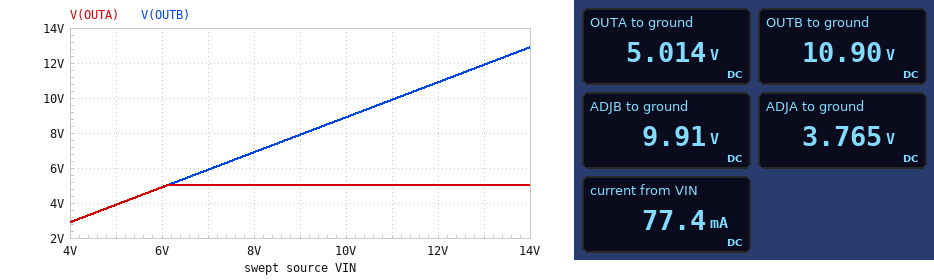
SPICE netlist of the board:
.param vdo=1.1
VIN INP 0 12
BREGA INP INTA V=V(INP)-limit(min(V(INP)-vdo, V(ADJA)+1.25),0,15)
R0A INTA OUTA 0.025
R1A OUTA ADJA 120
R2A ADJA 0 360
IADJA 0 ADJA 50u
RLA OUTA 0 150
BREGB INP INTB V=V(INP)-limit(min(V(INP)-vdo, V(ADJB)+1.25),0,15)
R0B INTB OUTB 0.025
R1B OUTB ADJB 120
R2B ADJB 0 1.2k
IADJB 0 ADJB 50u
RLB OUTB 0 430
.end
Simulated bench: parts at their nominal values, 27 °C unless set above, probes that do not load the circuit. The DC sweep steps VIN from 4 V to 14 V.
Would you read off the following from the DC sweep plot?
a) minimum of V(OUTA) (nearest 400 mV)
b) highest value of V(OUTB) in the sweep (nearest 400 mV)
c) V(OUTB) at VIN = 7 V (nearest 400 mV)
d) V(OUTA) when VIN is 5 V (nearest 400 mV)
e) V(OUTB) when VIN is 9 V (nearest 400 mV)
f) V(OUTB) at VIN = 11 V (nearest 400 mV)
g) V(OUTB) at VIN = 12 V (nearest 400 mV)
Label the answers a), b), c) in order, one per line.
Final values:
a) 2.8 V
b) 12.8 V
c) 6.0 V
d) 4.0 V
e) 8.0 V
f) 10.0 V
g) 10.8 V
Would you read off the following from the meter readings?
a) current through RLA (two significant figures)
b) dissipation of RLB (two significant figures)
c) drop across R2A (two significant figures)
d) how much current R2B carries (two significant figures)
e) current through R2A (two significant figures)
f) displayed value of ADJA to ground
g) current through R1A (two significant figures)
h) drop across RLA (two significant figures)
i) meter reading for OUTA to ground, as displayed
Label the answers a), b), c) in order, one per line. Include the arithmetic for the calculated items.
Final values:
a) (5.014 V) / 150 Ω = 33 mA
b) (10.9 V)^2 / 430 Ω = 280 mW
c) 3.765 V = 3.8 V
d) (9.91 V) / 1.2 kΩ = 8.3 mA
e) (3.765 V) / 360 Ω = 10 mA
f) 3.765 V
g) (5.014 V - 3.765 V) / 120 Ω = 10 mA
h) 5.014 V = 5.0 V
i) 5.014 V
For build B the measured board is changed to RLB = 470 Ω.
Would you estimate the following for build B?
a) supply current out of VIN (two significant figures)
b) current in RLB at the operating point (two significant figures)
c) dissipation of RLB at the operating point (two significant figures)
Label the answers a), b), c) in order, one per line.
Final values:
a) 75 mA
b) 23 mA
c) 250 mW
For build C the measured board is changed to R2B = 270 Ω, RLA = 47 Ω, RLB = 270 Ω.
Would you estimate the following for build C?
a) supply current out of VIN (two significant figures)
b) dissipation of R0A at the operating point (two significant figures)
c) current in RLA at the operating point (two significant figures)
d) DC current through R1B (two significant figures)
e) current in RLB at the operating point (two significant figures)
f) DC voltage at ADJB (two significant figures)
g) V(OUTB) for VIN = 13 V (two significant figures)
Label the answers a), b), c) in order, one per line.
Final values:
a) 140 mA
b) 340 µW
c) 110 mA
d) 10 mA
e) 15 mA
f) 2.8 V
g) 4.1 V
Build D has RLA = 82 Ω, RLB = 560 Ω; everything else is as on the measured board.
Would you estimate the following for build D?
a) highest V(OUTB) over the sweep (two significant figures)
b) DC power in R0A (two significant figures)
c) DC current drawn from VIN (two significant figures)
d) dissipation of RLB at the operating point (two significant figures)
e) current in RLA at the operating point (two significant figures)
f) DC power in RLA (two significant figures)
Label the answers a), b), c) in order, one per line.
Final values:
a) 13 V
b) 130 µW
c) 99 mA
d) 210 mW
e) 61 mA
f) 310 mW
